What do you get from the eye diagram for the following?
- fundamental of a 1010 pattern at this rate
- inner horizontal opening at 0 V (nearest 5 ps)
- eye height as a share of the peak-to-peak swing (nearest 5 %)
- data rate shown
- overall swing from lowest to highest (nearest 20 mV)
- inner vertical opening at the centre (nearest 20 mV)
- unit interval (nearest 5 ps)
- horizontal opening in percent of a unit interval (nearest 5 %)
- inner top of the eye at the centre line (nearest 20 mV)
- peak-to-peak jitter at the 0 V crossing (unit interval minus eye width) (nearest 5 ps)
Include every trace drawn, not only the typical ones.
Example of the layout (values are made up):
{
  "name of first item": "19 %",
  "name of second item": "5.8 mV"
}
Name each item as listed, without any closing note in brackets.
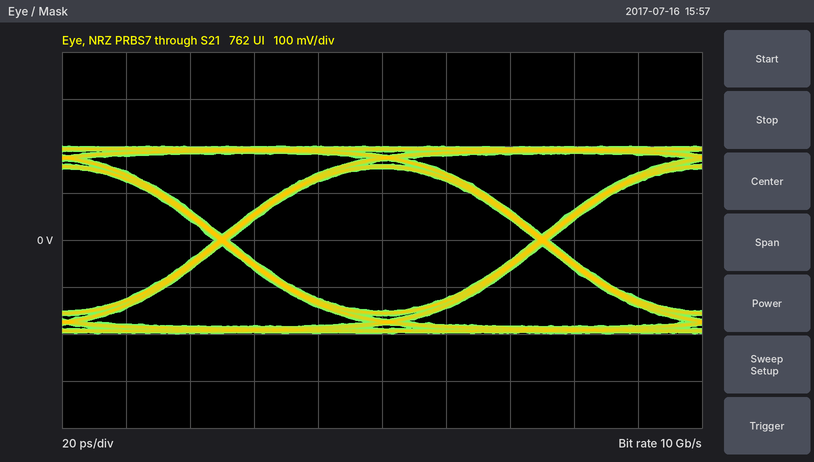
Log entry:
{
  "fundamental of a 1010 pattern at this rate": "5 GHz",
  "inner horizontal opening at 0 V": "95 ps",
  "eye height as a share of the peak-to-peak swing": "75 %",
  "data rate shown": "10 Gb/s",
  "overall swing from lowest to highest": "400 mV",
  "inner vertical opening at the centre": "300 mV",
  "unit interval": "100 ps",
  "horizontal opening in percent of a unit interval": "95 %",
  "inner top of the eye at the centre line": "160 mV",
  "peak-to-peak jitter at the 0 V crossing (unit interval minus eye width)": "5 ps"
}
